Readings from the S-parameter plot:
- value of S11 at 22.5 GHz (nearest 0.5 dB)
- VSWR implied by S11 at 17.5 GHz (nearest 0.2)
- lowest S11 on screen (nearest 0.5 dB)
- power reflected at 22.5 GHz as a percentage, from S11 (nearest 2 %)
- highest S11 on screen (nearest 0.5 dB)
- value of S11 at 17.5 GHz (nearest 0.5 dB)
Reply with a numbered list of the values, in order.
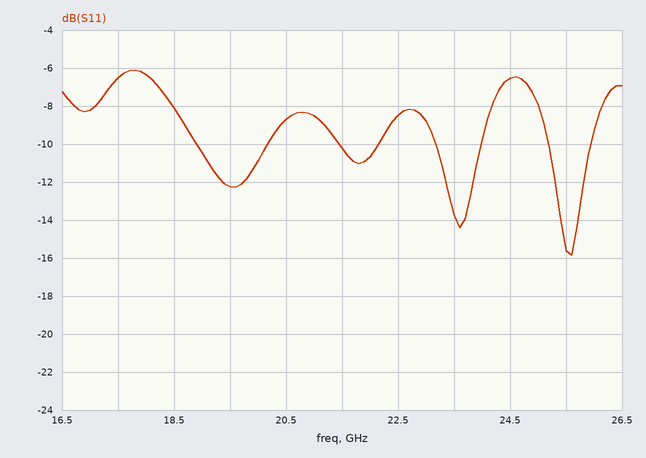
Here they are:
1. -8.5 dB
2. 2.8
3. -16.0 dB
4. 14 %
5. -6.0 dB
6. -6.5 dB
